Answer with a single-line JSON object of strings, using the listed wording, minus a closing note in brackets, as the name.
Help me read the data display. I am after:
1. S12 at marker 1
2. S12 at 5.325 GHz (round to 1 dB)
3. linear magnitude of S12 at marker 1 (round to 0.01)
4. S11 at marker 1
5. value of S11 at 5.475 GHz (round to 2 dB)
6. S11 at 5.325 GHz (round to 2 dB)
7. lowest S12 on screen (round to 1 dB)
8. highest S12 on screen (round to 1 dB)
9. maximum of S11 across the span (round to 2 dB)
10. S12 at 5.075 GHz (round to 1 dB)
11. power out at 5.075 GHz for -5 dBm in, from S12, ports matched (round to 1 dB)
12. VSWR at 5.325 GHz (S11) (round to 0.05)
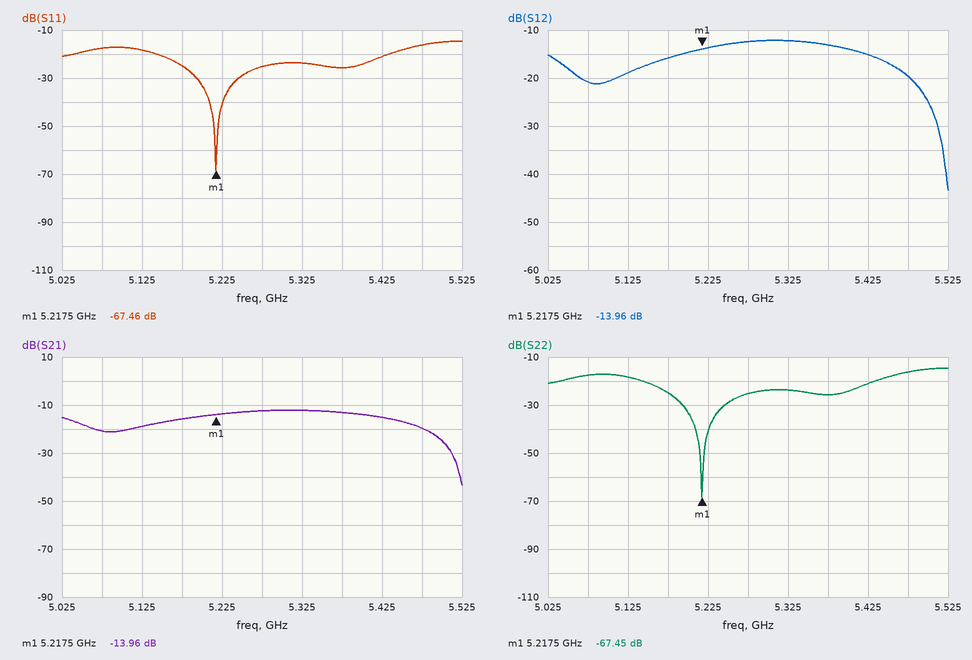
{"S12 at marker 1": "-13.96 dB", "S12 at 5.325 GHz": "-12 dB", "linear magnitude of S12 at marker 1": "0.20", "S11 at marker 1": "-67.46 dB", "value of S11 at 5.475 GHz": "-16 dB", "S11 at 5.325 GHz": "-24 dB", "lowest S12 on screen": "-43 dB", "highest S12 on screen": "-12 dB", "maximum of S11 across the span": "-14 dB", "S12 at 5.075 GHz": "-21 dB", "power out at 5.075 GHz for -5 dBm in, from S12, ports matched": "-26 dBm", "VSWR at 5.325 GHz (S11)": "1.15"}
